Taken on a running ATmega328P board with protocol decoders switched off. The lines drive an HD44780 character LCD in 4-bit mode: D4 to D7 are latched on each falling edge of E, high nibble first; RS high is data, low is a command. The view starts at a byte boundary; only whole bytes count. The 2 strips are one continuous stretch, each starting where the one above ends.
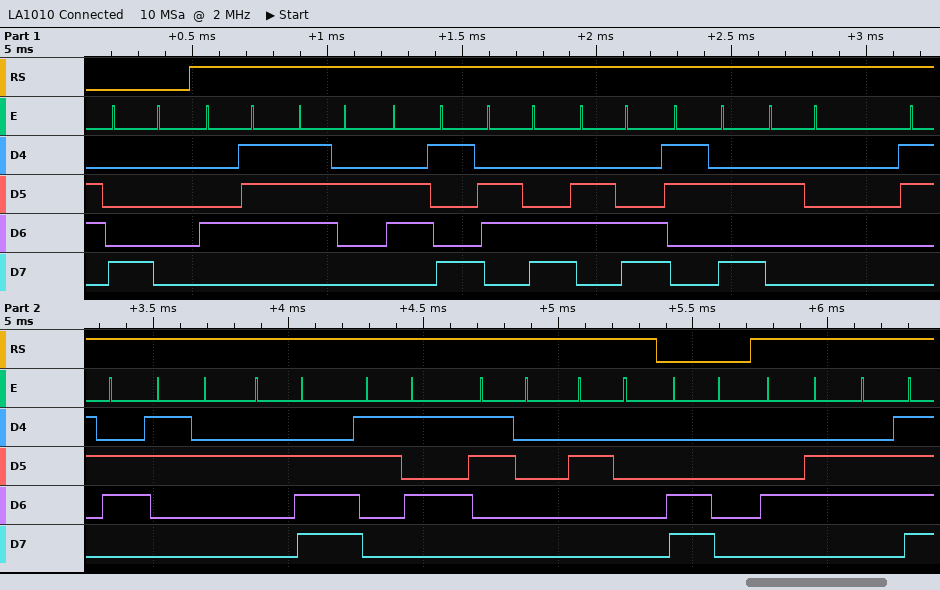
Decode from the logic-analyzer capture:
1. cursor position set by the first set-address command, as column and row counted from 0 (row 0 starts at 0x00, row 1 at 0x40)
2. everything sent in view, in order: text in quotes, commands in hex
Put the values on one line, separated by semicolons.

column 0, row 0; 0x80 "Grill: 62.50 " 0xC0 "Fo"
